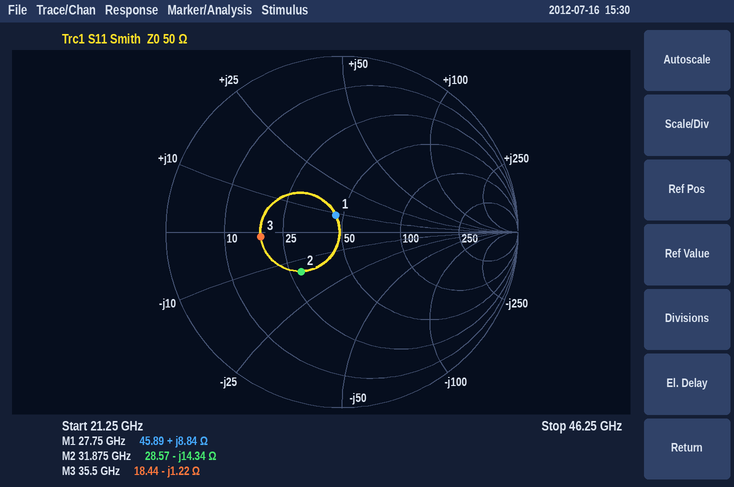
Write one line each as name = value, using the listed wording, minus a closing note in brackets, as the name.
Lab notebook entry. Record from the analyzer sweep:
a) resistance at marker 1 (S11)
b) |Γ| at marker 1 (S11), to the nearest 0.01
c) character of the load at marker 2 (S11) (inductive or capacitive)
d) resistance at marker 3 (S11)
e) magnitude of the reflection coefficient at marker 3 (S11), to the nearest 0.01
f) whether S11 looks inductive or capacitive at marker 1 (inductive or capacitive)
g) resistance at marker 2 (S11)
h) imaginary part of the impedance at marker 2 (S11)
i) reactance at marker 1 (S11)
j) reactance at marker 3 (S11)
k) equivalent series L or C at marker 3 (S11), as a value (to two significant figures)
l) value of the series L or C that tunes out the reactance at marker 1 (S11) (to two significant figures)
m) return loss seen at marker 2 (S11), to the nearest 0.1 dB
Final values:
resistance at marker 1 = 45.89 Ω
|Γ| at marker 1 (S11), to the nearest 0.01 = 0.10
character of the load at marker 2 (S11) = capacitive
resistance at marker 3 = 18.44 Ω
magnitude of the reflection coefficient at marker 3 (S11), to the nearest 0.01 = 0.46
whether S11 looks inductive or capacitive at marker 1 = inductive
resistance at marker 2 = 28.57 Ω
imaginary part of the impedance at marker 2 = -14.34 Ω
reactance at marker 1 = +8.84 Ω
reactance at marker 3 = -1.22 Ω
equivalent series L or C at marker 3 (S11), as a value = 3.7 pF
value of the series L or C that tunes out the reactance at marker 1 (S11) = 650 fF
return loss seen at marker 2 (S11), to the nearest 0.1 dB = 9.8 dB
